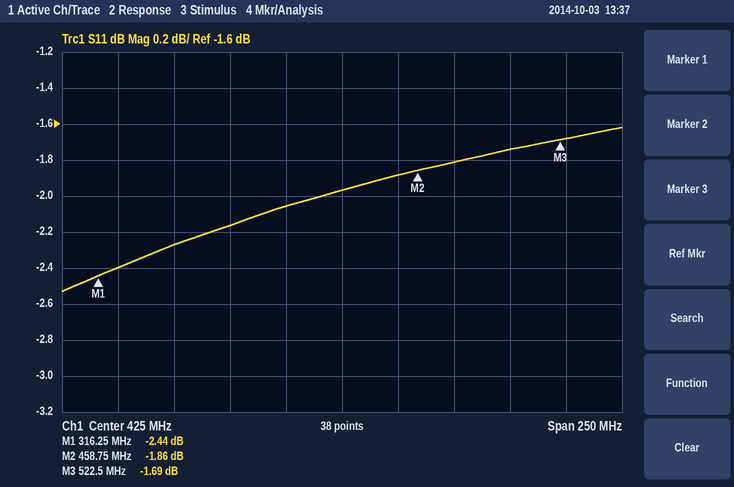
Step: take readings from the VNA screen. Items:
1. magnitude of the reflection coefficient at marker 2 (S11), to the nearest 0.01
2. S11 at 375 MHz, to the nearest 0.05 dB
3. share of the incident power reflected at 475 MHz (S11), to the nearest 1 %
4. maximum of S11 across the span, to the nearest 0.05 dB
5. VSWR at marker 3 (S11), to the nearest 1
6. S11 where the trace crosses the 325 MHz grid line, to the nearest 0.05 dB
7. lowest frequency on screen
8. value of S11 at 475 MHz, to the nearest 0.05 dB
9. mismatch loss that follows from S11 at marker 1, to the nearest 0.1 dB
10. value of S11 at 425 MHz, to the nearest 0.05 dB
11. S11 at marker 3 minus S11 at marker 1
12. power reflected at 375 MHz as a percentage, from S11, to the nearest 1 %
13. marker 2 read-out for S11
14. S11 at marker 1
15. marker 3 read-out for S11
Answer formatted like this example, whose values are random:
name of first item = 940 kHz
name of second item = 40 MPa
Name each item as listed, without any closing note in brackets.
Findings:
magnitude of the reflection coefficient at marker 2 (S11), to the nearest 0.01 = 0.81
S11 at 375 MHz, to the nearest 0.05 dB = -2.15 dB
share of the incident power reflected at 475 MHz (S11), to the nearest 1 % = 66 %
maximum of S11 across the span, to the nearest 0.05 dB = -1.60 dB
VSWR at marker 3 (S11), to the nearest 1 = 10
S11 where the trace crosses the 325 MHz grid line, to the nearest 0.05 dB = -2.40 dB
lowest frequency on screen = 300 MHz
value of S11 at 475 MHz, to the nearest 0.05 dB = -1.80 dB
mismatch loss that follows from S11 at marker 1, to the nearest 0.1 dB = 3.7 dB
value of S11 at 425 MHz, to the nearest 0.05 dB = -1.95 dB
S11 at marker 3 minus S11 at marker 1 = 0.75 dB
power reflected at 375 MHz as a percentage, from S11, to the nearest 1 % = 61 %
marker 2 read-out for S11 = -1.86 dB
S11 at marker 1 = -2.44 dB
marker 3 read-out for S11 = -1.69 dB
